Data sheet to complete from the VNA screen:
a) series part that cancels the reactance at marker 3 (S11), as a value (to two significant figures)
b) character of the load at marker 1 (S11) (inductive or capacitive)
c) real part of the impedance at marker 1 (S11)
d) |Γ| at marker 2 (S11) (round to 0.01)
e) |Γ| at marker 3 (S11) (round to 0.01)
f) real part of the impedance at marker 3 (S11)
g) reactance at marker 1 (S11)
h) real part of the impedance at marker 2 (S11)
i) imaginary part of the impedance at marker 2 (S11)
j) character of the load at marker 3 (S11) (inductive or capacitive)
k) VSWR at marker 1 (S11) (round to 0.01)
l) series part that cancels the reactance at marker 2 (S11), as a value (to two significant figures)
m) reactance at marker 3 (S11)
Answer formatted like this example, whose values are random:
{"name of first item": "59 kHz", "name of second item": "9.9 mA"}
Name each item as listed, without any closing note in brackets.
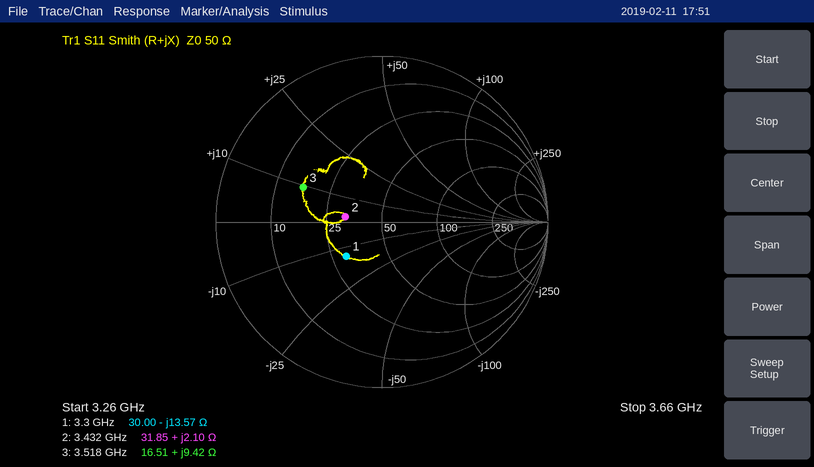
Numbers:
{"series part that cancels the reactance at marker 3 (S11), as a value": "4.8 pF", "character of the load at marker 1 (S11)": "capacitive", "real part of the impedance at marker 1": "30.00 Ω", "|Γ| at marker 2 (S11)": "0.22", "|Γ| at marker 3 (S11)": "0.52", "real part of the impedance at marker 3": "16.51 Ω", "reactance at marker 1": "-13.57 Ω", "real part of the impedance at marker 2": "31.85 Ω", "imaginary part of the impedance at marker 2": "+2.10 Ω", "character of the load at marker 3 (S11)": "inductive", "VSWR at marker 1 (S11)": "1.85", "series part that cancels the reactance at marker 2 (S11), as a value": "22 pF", "reactance at marker 3": "+9.42 Ω"}
